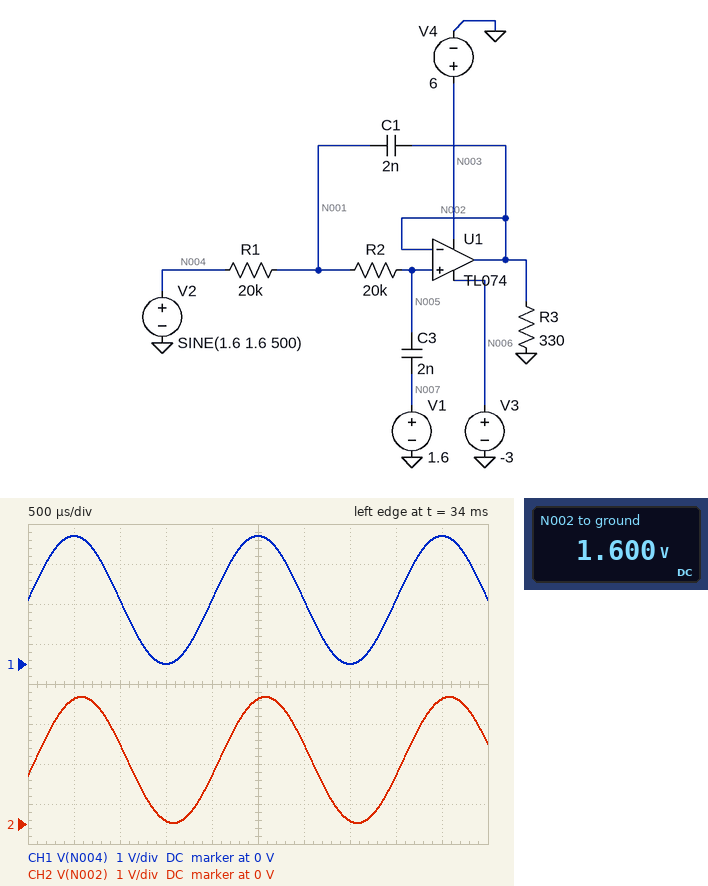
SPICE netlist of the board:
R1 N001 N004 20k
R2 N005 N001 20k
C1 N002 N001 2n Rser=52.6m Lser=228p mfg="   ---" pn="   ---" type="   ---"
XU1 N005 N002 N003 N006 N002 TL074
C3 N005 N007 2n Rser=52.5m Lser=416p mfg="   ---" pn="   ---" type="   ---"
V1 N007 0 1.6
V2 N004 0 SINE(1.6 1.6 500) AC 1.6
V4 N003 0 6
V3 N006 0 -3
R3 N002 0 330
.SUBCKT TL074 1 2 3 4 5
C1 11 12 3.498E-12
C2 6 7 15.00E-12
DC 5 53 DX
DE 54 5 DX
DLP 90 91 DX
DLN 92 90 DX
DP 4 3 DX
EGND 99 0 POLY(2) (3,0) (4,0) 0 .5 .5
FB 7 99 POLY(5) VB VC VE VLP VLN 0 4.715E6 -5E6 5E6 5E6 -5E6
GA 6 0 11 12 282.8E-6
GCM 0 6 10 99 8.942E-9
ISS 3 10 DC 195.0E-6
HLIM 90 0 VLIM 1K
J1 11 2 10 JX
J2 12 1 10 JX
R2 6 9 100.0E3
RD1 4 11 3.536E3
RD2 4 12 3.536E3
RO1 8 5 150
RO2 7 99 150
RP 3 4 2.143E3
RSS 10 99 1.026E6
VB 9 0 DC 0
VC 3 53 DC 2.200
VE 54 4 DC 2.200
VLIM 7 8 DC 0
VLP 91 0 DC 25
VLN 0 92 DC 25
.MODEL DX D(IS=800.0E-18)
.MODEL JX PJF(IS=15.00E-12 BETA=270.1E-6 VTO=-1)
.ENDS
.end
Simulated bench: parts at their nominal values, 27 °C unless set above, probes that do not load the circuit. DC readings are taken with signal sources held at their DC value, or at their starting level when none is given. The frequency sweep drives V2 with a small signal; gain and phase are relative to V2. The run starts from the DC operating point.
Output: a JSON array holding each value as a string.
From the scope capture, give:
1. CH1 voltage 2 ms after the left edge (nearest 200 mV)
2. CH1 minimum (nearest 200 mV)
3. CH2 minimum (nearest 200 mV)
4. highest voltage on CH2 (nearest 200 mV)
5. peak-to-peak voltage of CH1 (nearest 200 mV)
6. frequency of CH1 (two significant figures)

["1.6 V", "0 V", "0 V", "3.2 V", "3.2 V", "500 Hz"]
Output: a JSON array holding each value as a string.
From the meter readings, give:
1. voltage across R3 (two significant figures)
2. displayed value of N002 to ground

["1.6 V", "1.600 V"]
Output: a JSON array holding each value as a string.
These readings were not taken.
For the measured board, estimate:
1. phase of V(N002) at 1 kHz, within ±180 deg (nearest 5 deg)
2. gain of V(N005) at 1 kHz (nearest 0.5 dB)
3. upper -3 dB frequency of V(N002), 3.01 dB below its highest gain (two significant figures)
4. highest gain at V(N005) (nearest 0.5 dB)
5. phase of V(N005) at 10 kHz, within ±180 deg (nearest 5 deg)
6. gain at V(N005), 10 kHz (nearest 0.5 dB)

["-30 deg", "-0.5 dB", "2.6 kHz", "0 dB", "-135 deg", "-17.5 dB"]
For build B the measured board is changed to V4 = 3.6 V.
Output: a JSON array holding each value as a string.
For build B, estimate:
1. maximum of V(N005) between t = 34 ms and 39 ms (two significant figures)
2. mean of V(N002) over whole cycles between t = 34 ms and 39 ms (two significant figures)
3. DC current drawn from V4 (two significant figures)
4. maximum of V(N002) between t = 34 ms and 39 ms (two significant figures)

["3.1 V", "1.3 V", "3.3 mA", "2.1 V"]
